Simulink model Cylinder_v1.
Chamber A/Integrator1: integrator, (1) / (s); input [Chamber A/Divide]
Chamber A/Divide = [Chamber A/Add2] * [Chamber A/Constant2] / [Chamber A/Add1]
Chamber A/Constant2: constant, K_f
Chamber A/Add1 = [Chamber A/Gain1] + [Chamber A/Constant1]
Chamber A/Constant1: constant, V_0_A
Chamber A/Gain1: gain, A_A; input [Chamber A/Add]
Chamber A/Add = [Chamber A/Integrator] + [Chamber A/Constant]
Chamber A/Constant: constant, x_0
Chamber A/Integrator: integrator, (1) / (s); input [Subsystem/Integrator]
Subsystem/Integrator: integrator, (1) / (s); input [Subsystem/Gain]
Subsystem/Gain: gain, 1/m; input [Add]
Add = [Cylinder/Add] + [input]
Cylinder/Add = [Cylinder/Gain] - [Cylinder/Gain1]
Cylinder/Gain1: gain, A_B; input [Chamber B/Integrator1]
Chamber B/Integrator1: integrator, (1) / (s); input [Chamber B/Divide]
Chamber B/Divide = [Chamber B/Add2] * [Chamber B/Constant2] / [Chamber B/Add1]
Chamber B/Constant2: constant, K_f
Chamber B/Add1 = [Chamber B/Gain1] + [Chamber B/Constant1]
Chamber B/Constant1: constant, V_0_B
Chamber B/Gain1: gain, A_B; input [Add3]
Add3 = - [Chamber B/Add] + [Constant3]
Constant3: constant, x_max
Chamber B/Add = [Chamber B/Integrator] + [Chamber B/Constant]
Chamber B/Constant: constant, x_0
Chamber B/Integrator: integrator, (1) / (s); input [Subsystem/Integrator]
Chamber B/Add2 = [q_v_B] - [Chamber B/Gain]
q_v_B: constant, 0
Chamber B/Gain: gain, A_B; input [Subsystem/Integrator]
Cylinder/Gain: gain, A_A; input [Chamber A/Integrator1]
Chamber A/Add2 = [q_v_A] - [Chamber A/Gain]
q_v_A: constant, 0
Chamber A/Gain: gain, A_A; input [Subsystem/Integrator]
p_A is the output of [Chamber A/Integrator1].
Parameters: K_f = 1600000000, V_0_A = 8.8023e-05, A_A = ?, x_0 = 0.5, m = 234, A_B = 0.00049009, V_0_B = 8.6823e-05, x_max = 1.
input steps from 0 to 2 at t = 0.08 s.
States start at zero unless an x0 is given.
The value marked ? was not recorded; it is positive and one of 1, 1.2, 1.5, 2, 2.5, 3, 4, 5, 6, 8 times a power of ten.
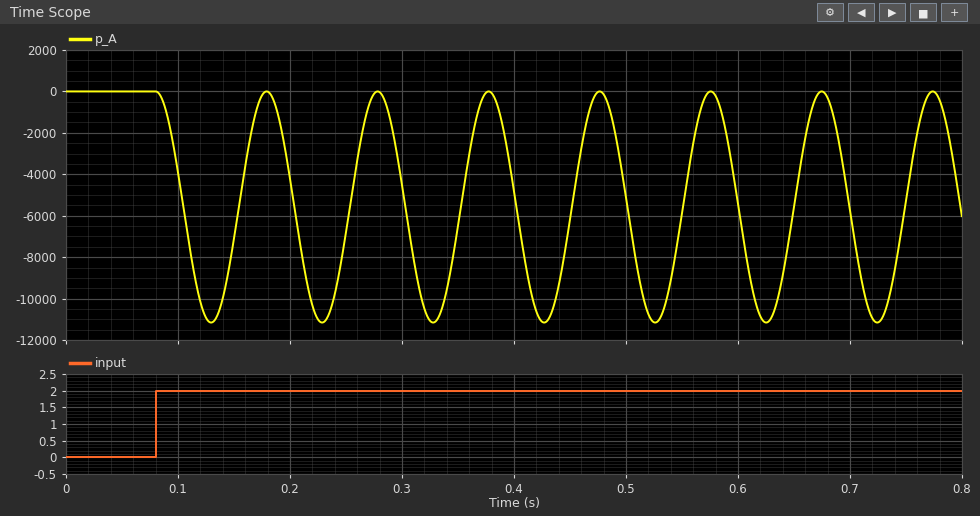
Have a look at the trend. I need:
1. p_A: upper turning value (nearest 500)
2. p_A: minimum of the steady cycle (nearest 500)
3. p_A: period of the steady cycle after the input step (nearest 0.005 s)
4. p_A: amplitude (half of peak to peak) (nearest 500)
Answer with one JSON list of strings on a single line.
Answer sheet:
["0", "-11000", "0.100 s", "5500"]
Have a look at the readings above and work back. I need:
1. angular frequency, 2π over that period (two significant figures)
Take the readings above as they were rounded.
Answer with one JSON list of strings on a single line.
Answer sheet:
["63 rad/s"]
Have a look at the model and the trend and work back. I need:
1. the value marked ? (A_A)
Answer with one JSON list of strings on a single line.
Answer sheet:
["0.0008"]
